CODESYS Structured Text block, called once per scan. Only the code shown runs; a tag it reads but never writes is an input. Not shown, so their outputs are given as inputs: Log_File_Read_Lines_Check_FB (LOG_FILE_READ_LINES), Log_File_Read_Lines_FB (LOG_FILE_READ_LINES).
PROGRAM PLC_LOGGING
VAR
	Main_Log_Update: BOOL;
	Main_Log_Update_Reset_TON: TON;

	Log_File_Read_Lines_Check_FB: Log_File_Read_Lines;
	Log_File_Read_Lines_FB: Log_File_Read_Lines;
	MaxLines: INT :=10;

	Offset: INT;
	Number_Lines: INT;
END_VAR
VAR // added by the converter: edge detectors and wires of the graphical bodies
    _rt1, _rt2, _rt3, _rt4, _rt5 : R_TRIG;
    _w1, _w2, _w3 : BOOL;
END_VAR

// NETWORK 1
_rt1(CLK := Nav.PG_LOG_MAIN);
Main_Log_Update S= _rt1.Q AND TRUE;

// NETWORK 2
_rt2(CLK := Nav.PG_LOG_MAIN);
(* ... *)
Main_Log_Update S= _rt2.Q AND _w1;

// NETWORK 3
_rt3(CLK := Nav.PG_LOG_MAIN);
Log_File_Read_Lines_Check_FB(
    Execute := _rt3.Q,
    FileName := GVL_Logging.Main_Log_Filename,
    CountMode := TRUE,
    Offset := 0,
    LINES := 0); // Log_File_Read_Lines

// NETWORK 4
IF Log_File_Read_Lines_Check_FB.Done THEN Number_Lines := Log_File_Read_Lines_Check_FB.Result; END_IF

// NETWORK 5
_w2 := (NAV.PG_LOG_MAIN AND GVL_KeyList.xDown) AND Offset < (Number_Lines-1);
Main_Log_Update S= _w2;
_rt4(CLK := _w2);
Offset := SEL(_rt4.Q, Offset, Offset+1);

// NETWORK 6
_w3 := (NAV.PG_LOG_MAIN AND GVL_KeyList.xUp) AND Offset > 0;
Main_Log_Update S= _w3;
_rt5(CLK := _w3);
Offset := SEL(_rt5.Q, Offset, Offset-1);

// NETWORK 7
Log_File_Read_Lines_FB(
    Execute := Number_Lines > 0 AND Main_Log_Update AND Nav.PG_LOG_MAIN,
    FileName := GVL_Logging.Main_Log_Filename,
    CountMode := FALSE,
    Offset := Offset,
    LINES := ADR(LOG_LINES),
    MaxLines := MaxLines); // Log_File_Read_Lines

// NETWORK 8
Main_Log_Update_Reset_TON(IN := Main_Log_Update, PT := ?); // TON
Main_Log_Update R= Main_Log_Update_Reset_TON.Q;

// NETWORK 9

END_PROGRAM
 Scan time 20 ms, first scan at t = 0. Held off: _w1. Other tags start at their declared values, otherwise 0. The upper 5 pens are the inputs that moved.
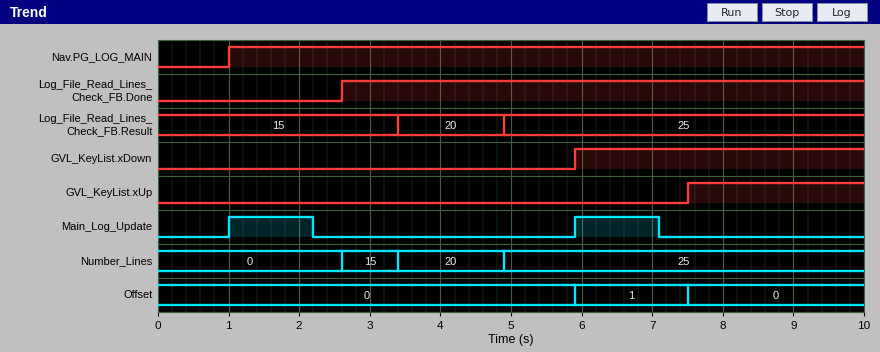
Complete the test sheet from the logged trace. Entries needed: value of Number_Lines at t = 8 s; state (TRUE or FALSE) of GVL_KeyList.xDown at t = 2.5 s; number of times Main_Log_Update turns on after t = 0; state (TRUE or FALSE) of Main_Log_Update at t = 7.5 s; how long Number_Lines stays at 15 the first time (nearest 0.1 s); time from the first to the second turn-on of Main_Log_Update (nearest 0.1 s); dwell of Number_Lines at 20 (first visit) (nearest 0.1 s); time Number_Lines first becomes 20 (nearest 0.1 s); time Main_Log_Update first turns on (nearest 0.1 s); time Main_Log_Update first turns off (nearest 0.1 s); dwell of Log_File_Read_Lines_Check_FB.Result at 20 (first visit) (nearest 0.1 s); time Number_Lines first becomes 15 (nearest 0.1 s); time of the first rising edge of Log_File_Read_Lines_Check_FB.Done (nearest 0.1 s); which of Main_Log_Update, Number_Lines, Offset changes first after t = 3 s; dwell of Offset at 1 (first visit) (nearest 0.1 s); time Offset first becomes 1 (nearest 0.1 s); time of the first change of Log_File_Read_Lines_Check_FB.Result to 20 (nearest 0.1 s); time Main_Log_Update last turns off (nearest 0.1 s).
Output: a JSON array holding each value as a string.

["25", "FALSE", "2", "FALSE", "0.8 s", "4.9 s", "1.5 s", "3.4 s", "1.0 s", "2.2 s", "1.5 s", "2.6 s", "2.6 s", "Number_Lines", "1.6 s", "5.9 s", "3.4 s", "7.1 s"]
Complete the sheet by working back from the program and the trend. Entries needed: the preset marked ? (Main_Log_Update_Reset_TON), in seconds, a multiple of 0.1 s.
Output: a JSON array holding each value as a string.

["1.2 s"]
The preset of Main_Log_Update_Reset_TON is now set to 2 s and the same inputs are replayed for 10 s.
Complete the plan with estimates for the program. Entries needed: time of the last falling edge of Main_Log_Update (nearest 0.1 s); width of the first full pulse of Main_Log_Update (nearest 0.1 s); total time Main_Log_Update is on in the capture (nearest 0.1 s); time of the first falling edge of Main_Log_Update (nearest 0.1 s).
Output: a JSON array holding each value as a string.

["7.9 s", "2.0 s", "4.0 s", "3.0 s"]
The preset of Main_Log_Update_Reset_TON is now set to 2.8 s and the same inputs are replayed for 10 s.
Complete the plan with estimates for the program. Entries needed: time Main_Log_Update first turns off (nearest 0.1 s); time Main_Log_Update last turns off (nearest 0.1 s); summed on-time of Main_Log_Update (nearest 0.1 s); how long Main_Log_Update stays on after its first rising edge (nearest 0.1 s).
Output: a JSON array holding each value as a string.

["3.8 s", "8.7 s", "5.6 s", "2.8 s"]
